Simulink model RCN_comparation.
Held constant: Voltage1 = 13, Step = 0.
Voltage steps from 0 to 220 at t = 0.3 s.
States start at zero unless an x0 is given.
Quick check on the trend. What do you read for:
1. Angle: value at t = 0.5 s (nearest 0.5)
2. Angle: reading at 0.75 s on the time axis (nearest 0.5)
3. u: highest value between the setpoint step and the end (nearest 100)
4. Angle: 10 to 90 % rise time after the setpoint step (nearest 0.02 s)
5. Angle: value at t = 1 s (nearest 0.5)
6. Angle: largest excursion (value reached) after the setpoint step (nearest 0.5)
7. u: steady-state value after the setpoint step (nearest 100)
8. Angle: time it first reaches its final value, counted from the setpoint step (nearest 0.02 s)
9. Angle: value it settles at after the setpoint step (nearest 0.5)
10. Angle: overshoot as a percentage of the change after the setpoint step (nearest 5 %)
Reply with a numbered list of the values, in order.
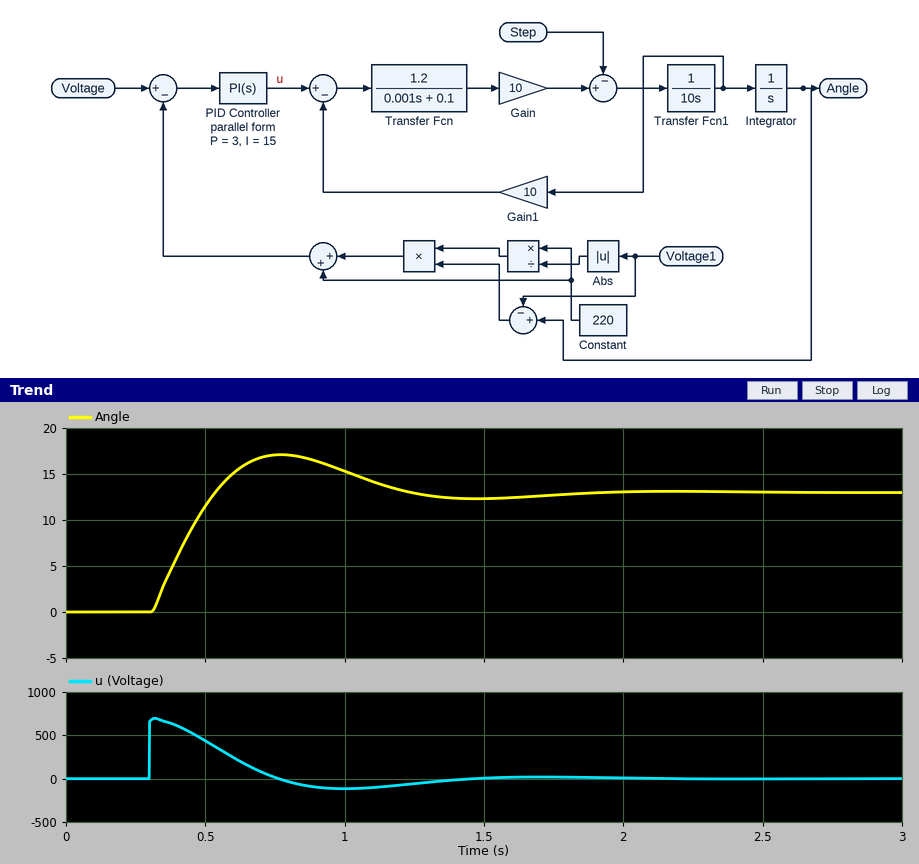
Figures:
1. 11.5
2. 17.0
3. 700
4. 0.18 s
5. 15.5
6. 17.0
7. 0
8. 0.24 s
9. 13.0
10. 30 %
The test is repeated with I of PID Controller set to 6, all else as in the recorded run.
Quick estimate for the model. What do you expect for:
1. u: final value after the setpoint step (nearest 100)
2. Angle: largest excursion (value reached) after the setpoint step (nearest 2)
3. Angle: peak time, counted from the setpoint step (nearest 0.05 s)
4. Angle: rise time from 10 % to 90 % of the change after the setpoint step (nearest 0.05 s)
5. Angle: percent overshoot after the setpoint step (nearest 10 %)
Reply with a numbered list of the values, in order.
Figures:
1. 0
2. 16
3. 0.65 s
4. 0.25 s
5. 20 %
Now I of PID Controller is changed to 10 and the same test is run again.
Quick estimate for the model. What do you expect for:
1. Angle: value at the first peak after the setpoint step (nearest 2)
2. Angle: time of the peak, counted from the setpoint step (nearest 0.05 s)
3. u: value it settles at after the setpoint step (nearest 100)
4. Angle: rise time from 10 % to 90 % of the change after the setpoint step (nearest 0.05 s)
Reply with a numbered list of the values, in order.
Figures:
1. 16
2. 0.55 s
3. 0
4. 0.20 s
